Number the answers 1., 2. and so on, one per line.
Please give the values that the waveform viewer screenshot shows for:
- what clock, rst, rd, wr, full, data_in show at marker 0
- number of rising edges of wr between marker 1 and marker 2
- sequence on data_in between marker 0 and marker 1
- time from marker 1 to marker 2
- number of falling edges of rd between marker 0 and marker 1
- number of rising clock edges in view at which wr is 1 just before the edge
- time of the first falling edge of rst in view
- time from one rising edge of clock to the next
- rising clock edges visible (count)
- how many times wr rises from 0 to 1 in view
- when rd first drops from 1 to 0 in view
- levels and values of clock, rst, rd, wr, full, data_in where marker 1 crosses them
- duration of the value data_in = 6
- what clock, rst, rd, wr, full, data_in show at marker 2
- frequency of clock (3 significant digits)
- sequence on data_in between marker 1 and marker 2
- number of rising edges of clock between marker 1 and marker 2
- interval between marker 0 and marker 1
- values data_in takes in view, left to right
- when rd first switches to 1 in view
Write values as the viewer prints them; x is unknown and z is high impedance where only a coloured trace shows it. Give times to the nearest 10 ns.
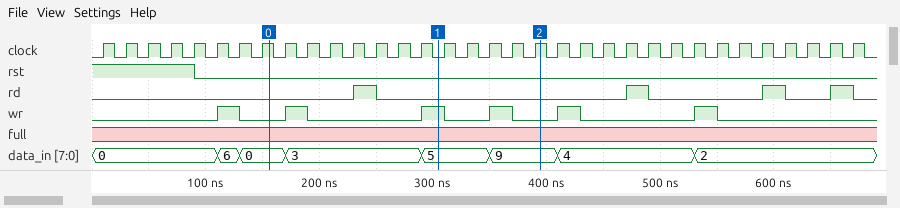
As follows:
1. clock=1, rst=0, rd=0, wr=0, full=x, data_in=0
2. 1
3. 0, 3, 5
4. 90 ns
5. 1
6. 6
7. 90 ns
8. 20 ns
9. 34
10. 6
11. 250 ns
12. clock=0, rst=0, rd=0, wr=1, full=x, data_in=5
13. 20 ns
14. clock=1, rst=0, rd=0, wr=0, full=x, data_in=9
15. 50.0 MHz
16. 5, 9
17. 5
18. 150 ns
19. 0, 6, 0, 3, 5, 9, 4, 2
20. 230 ns
